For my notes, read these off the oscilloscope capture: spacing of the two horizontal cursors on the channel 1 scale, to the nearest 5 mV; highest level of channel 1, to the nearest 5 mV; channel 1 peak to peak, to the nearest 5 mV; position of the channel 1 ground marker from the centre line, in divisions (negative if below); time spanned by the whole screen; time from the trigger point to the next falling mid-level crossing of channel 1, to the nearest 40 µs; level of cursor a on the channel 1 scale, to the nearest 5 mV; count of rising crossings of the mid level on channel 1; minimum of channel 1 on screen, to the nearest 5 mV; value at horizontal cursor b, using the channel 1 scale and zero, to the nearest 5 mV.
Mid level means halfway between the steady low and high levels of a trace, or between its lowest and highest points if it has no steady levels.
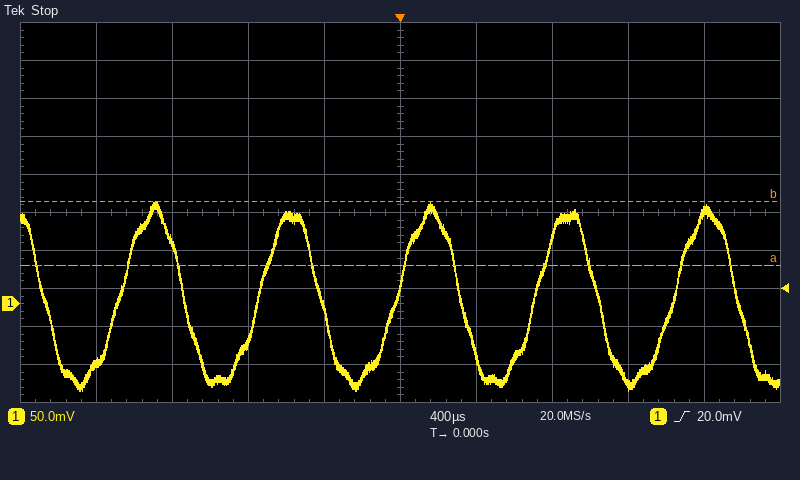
85 mV
135 mV
250 mV
-2.4 div
4 ms
320 µs
50 mV
5
-115 mV
135 mV
